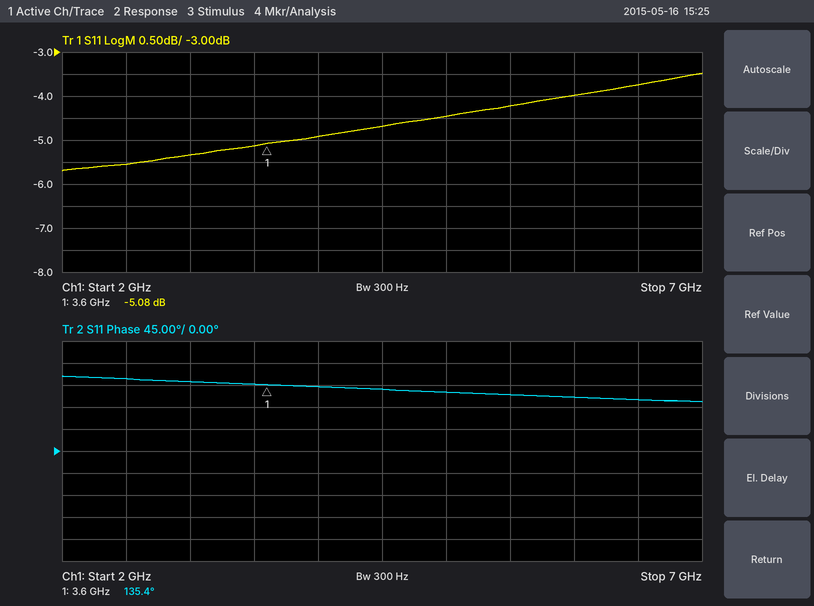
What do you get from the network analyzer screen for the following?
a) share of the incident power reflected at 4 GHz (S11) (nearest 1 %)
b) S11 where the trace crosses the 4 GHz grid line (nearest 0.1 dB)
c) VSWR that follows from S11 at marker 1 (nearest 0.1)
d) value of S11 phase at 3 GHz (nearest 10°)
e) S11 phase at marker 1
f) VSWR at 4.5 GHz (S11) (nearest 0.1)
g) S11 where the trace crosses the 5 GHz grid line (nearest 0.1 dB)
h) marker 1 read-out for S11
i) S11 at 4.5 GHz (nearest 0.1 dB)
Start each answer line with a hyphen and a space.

- 32 %
- -4.9 dB
- 3.5
- 140°
- 135.4°
- 3.8
- -4.5 dB
- -5.08 dB
- -4.7 dB
